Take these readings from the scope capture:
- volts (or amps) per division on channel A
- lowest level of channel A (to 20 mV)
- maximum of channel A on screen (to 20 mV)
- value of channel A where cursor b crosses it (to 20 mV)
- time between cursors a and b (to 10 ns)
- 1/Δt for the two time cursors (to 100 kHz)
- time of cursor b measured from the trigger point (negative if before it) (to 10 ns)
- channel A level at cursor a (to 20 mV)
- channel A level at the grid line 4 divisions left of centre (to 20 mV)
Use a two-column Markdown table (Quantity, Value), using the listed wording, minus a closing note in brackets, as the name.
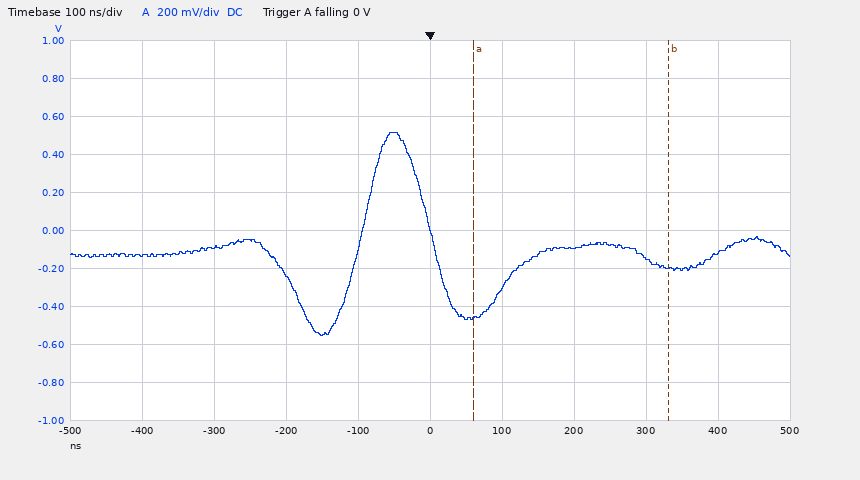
| Quantity | Value |
|---|---|
| volts (or amps) per division on channel A | 200 mV |
| lowest level of channel A | -560 mV |
| maximum of channel A on screen | 520 mV |
| value of channel A where cursor b crosses it | -200 mV |
| time between cursors a and b | 270 ns |
| 1/Δt for the two time cursors | 3.7 MHz |
| time of cursor b measured from the trigger point (negative if before it) | +330 ns |
| channel A level at cursor a | -460 mV |
| channel A level at the grid line 4 divisions left of centre | -140 mV |
